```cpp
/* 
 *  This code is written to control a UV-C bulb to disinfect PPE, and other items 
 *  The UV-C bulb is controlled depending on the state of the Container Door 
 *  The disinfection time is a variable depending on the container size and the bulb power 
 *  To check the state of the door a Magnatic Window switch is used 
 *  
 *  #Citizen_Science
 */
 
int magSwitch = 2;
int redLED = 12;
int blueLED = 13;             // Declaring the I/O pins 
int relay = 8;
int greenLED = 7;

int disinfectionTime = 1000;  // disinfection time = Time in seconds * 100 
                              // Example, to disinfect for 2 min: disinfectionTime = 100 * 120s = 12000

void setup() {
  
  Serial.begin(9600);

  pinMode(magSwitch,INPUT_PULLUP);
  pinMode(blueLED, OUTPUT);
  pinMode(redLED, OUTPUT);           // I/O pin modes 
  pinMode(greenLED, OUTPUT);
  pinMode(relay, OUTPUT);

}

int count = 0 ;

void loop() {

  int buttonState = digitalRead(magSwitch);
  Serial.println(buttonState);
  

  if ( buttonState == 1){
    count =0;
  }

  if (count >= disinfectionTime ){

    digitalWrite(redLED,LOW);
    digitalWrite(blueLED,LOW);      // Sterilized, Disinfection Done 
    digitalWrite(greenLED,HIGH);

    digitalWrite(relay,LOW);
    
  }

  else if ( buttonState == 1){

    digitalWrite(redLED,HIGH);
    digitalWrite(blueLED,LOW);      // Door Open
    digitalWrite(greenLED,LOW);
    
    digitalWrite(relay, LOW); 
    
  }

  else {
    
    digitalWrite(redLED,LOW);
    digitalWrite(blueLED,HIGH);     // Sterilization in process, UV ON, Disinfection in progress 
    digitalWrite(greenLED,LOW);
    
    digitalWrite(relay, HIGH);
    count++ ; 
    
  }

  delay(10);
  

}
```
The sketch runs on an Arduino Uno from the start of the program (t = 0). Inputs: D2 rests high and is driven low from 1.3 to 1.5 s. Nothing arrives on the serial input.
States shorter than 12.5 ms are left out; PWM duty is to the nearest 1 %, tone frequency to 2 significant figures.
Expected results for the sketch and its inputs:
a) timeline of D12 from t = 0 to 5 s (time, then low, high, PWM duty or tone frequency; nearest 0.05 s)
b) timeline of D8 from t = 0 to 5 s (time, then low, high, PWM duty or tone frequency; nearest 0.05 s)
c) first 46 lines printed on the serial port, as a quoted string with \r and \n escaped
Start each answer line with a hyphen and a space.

- 0 s high; 1.3 s low; 1.5 s high
- 0 s low; 1.3 s high; 1.5 s low
- "1\r\n1\r\n1\r\n1\r\n1\r\n1\r\n1\r\n1\r\n1\r\n1\r\n1\r\n1\r\n1\r\n1\r\n1\r\n1\r\n1\r\n1\r\n1\r\n1\r\n1\r\n1\r\n1\r\n1\r\n1\r\n1\r\n1\r\n1\r\n1\r\n1\r\n1\r\n1\r\n1\r\n1\r\n1\r\n1\r\n1\r\n1\r\n1\r\n1\r\n1\r\n1\r\n1\r\n1\r\n1\r\n1\r\n"
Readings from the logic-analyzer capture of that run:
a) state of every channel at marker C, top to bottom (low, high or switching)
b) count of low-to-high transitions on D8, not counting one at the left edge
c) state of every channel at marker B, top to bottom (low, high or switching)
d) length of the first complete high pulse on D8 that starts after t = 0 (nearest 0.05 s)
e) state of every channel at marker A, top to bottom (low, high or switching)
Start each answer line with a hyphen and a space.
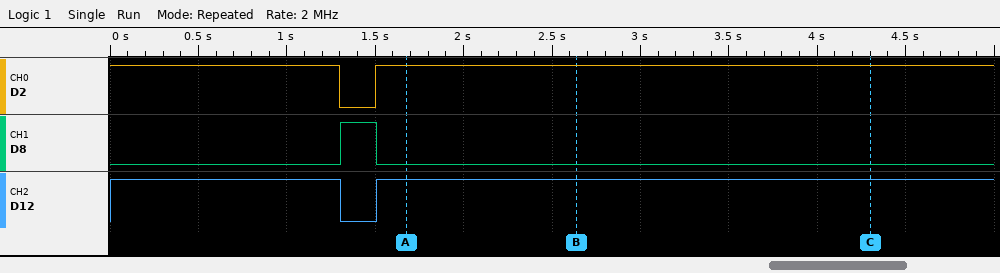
- D2 high, D8 low, D12 high
- 1
- D2 high, D8 low, D12 high
- 0.20 s
- D2 high, D8 low, D12 high
